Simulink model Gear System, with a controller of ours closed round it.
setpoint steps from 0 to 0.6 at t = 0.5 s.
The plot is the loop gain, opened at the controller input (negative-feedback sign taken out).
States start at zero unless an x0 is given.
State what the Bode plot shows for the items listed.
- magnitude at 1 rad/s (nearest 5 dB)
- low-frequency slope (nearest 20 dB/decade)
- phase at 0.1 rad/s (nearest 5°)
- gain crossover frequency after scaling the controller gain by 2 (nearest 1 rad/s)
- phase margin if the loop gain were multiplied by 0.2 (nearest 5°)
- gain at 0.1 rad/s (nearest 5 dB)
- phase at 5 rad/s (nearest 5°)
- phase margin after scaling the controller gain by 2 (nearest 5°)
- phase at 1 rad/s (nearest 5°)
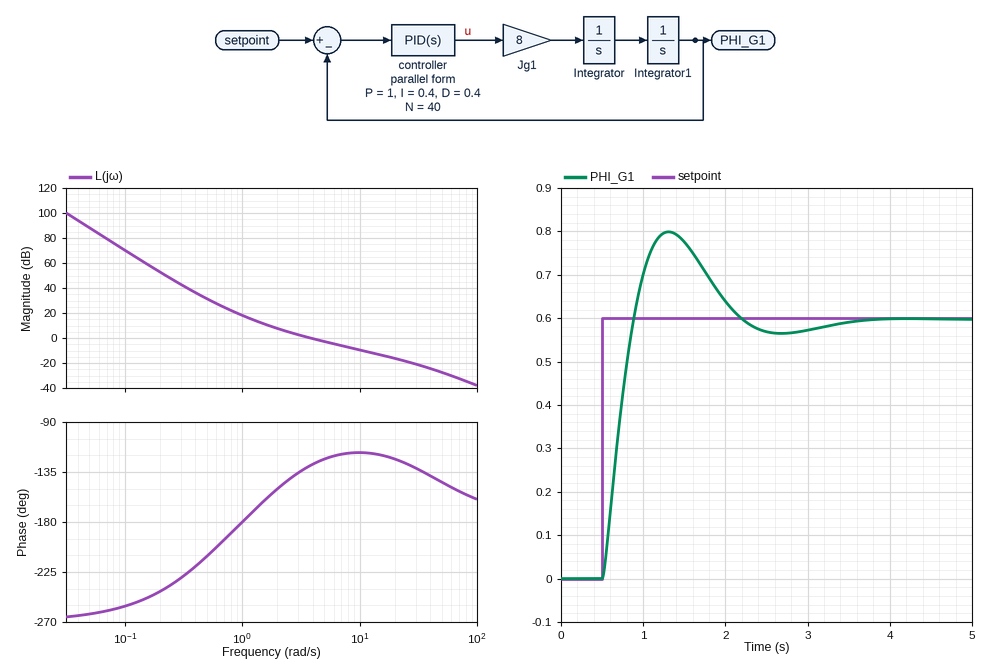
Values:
20 dB
-60 dB/decade
-255°
7 rad/s
10°
70 dB
-125°
60°
-180°
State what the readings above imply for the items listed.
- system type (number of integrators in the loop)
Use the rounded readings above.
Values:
3
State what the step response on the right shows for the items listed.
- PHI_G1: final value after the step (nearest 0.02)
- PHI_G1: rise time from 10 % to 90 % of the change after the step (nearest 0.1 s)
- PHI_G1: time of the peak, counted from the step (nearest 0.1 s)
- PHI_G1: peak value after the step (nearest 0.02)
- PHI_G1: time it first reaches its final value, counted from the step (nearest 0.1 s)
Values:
0.60
0.3 s
0.8 s
0.80
0.4 s
